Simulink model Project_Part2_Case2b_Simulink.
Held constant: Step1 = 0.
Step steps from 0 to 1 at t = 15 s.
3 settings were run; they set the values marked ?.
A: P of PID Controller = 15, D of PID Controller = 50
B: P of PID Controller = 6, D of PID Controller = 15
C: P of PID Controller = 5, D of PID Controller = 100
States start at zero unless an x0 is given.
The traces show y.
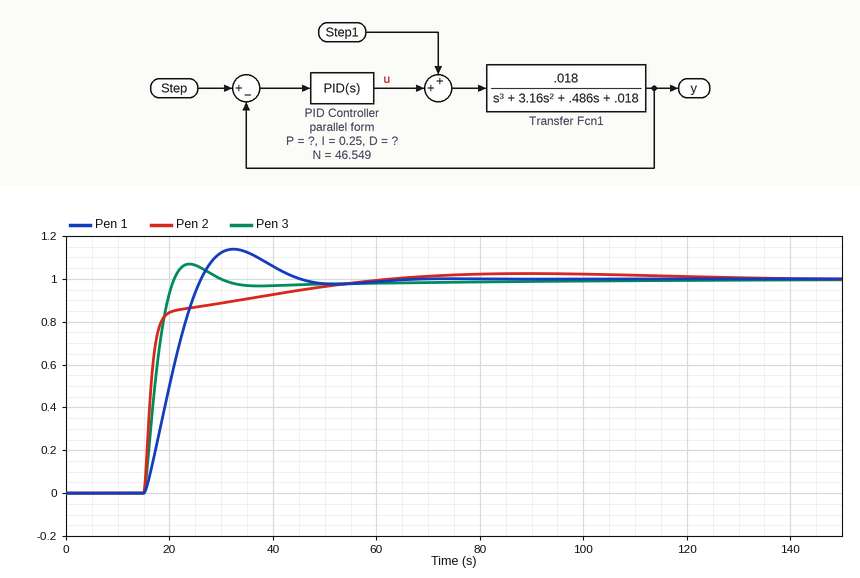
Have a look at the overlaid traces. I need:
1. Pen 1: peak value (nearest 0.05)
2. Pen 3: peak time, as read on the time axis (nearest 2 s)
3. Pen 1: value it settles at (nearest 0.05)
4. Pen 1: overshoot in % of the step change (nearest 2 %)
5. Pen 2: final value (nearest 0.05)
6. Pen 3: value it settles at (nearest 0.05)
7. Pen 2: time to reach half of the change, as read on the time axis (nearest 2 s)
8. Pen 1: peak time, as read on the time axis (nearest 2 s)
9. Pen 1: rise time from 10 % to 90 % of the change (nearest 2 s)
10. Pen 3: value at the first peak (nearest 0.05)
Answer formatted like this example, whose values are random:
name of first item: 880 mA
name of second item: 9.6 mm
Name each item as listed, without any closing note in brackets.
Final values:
Pen 1: peak value: 1.15
Pen 3: peak time, as read on the time axis: 24 s
Pen 1: value it settles at: 1.00
Pen 1: overshoot in % of the step change: 14 %
Pen 2: final value: 1.00
Pen 3: value it settles at: 1.00
Pen 2: time to reach half of the change, as read on the time axis: 16 s
Pen 1: peak time, as read on the time axis: 32 s
Pen 1: rise time from 10 % to 90 % of the change: 8 s
Pen 3: value at the first peak: 1.05
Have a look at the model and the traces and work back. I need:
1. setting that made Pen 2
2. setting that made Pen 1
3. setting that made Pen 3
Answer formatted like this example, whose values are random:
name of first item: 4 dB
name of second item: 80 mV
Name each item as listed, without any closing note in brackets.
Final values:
setting that made Pen 2: C
setting that made Pen 1: B
setting that made Pen 3: A
